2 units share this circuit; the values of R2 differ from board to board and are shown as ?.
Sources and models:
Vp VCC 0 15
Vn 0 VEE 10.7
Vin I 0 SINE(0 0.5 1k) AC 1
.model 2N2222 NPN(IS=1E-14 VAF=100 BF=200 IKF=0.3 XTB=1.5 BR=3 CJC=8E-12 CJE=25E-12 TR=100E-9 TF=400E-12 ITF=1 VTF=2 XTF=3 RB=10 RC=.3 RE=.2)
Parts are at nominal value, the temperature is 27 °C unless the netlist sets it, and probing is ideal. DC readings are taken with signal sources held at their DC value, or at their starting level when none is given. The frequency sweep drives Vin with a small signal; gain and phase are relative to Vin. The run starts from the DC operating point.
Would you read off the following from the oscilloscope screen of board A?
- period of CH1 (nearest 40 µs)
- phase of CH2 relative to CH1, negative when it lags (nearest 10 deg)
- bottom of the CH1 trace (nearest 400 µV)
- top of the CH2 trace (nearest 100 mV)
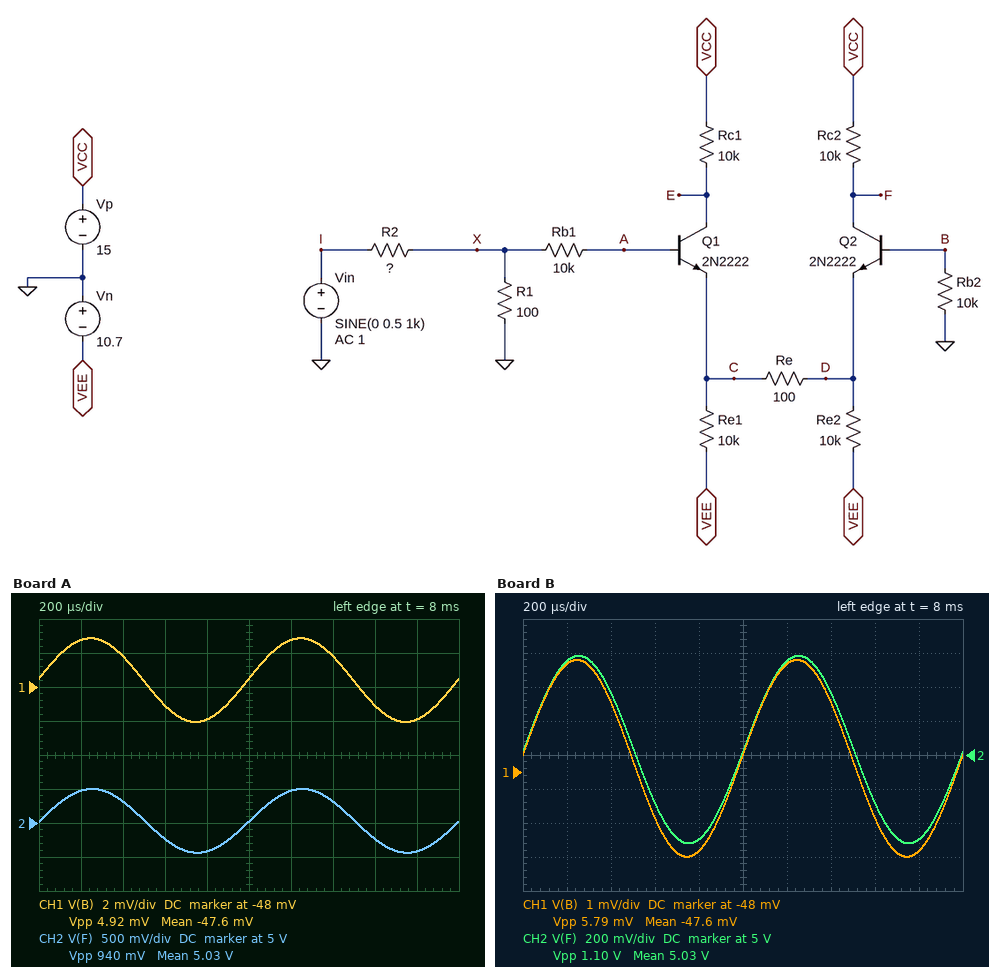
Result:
1.00 ms
0 deg
-50.0 mV
5.5 V
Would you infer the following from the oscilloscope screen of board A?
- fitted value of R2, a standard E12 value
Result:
3.9 kΩ
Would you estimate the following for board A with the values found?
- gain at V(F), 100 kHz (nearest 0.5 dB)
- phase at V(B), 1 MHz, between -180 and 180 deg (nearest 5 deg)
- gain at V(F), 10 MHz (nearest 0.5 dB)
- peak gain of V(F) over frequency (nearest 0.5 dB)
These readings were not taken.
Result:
-8.0 dB
-20 deg
-47.5 dB
-0.5 dB
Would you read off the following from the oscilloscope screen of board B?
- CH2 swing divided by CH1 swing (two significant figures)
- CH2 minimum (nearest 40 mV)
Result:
190
4.48 V
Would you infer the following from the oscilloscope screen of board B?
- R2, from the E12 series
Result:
3.3 kΩ
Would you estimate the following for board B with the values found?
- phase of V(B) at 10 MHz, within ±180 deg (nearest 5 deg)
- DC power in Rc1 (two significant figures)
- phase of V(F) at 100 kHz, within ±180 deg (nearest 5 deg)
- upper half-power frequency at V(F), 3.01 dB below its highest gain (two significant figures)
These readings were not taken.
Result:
-15 deg
9.9 mW
-65 deg
48 kHz
